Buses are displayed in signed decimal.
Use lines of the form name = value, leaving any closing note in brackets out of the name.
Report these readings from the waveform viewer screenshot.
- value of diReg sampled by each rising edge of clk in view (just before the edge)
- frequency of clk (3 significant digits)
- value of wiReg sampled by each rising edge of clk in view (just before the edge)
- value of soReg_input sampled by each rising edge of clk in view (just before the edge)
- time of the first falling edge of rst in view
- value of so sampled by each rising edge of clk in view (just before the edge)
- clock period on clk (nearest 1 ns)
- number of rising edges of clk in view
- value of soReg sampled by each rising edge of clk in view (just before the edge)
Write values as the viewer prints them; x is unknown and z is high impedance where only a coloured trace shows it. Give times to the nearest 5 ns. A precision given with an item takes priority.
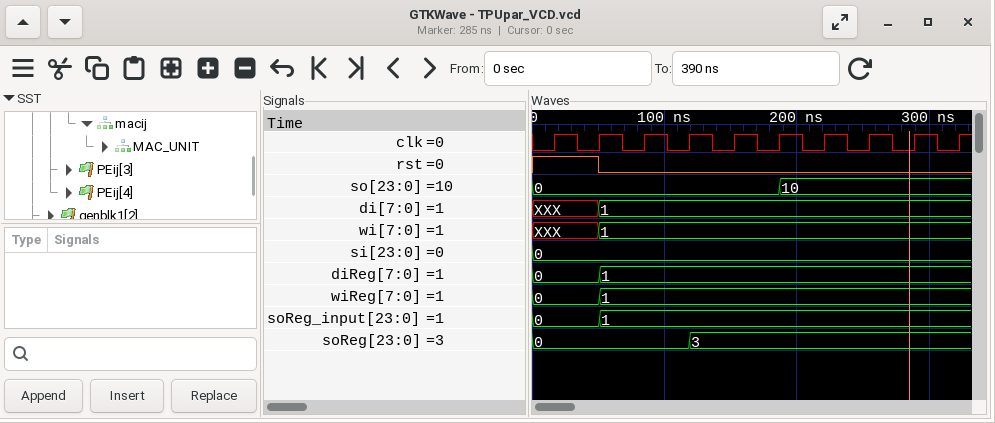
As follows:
value of diReg sampled by each rising edge of clk in view = 0, 0, 1, 1, 1, 1, 1, 1, 1, 1
frequency of clk = 29.4 MHz
value of wiReg sampled by each rising edge of clk in view = 0, 0, 1, 1, 1, 1, 1, 1, 1, 1
value of soReg_input sampled by each rising edge of clk in view = 0, 0, 1, 1, 1, 1, 1, 1, 1, 1
time of the first falling edge of rst in view = 50 ns
value of so sampled by each rising edge of clk in view = 0, 0, 0, 0, 0, 0, 10, 10, 10, 10
clock period on clk = 34 ns
number of rising edges of clk in view = 10
value of soReg sampled by each rising edge of clk in view = 0, 0, 0, 0, 3, 3, 3, 3, 3, 3
